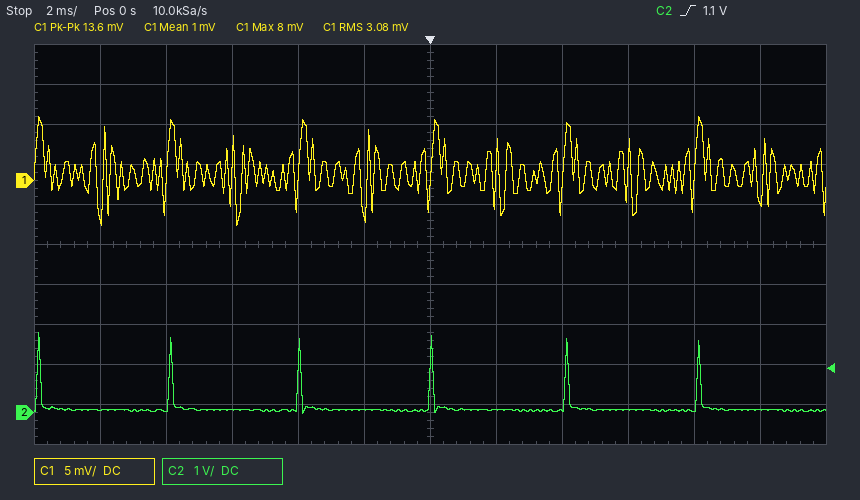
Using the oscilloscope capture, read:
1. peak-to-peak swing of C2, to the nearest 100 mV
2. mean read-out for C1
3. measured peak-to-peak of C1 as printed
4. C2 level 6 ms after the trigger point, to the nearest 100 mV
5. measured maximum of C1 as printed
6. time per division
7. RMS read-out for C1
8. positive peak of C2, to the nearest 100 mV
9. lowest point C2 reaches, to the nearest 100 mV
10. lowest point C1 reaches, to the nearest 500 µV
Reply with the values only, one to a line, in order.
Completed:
2.0 V
1 mV
13.6 mV
100 mV
8 mV
2 ms
3.08 mV
2.0 V
0.0 V
-5.5 mV
